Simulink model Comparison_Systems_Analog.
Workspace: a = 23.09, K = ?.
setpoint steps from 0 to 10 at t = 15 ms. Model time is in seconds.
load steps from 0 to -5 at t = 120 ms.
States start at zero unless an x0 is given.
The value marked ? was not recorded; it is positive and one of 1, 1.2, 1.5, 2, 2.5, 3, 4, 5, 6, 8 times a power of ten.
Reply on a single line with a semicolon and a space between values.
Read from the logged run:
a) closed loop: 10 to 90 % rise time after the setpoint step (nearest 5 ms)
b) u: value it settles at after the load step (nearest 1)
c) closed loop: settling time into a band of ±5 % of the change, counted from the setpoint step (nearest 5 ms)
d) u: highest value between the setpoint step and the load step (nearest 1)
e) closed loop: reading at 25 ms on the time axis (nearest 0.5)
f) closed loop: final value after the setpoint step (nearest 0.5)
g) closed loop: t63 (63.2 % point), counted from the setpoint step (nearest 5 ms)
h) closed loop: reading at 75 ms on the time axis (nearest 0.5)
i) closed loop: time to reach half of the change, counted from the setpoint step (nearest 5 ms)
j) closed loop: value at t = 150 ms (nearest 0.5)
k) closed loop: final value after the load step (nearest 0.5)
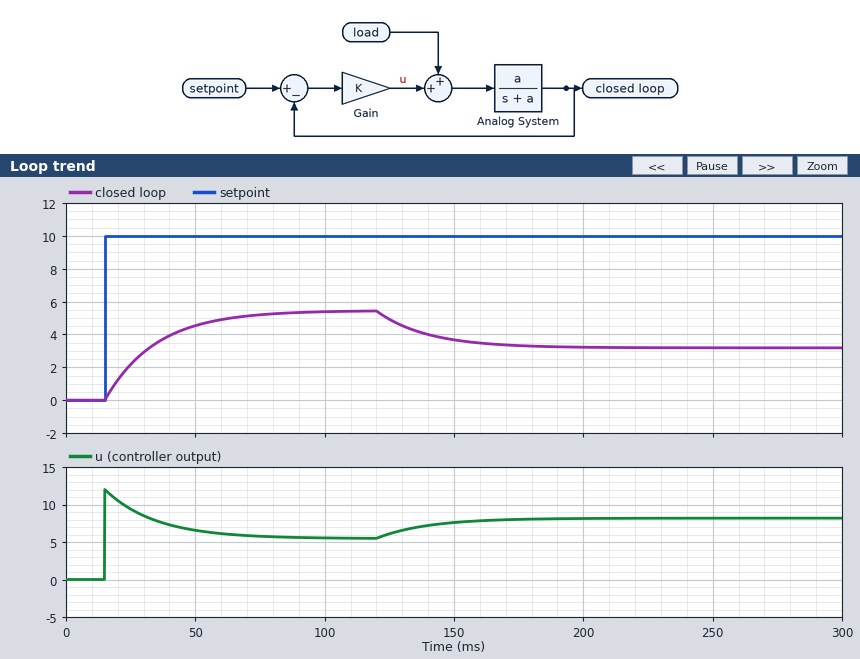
45 ms; 8; 60 ms; 12; 2.0; 5.5; 20 ms; 5.0; 15 ms; 3.5; 3.0
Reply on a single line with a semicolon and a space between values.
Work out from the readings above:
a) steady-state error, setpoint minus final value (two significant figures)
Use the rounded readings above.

4.5
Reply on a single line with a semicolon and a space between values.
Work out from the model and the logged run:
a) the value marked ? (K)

1.2
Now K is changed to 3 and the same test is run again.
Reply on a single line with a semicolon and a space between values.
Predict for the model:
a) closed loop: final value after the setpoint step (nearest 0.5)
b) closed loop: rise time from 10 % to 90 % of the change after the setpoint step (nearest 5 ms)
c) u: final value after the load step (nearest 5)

7.5; 25 ms; 10
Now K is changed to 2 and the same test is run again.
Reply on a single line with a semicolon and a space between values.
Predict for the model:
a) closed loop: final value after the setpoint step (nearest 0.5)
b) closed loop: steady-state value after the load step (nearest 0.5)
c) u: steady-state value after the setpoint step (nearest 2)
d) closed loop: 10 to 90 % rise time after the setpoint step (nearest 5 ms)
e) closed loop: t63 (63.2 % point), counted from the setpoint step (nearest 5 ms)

6.5; 5.0; 6; 30 ms; 15 ms
